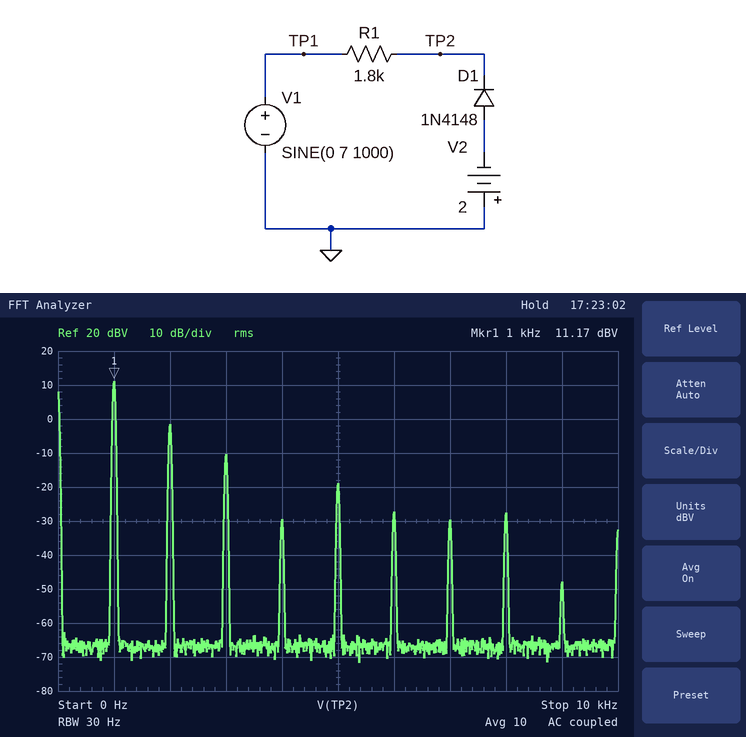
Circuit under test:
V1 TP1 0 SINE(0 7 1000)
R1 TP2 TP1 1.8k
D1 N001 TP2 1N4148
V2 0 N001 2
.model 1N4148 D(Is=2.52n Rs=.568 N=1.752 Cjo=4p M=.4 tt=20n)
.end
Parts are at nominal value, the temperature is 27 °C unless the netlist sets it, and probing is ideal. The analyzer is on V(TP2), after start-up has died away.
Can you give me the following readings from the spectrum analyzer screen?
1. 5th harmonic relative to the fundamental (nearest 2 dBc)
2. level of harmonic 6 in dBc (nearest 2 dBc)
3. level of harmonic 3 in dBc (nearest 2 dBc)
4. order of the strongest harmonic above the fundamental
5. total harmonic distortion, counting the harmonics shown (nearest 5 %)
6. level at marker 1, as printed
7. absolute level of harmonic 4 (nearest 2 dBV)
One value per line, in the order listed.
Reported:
-30 dBc
-38 dBc
-22 dBc
2
25 %
11.17 dBV
-30 dBV
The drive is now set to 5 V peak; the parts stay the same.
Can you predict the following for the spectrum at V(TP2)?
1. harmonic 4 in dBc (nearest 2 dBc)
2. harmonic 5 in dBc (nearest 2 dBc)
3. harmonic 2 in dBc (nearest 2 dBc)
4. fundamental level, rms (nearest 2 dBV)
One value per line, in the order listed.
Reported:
-36 dBc
-36 dBc
-16 dBc
10 dBV
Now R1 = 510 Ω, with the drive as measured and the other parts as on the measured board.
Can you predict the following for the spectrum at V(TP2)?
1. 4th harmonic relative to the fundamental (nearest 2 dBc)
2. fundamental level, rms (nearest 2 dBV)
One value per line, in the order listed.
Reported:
-42 dBc
12 dBV
